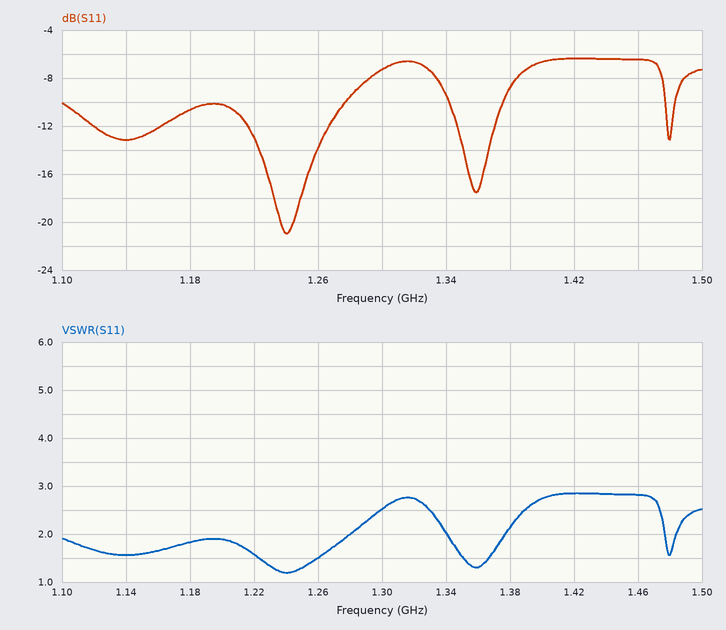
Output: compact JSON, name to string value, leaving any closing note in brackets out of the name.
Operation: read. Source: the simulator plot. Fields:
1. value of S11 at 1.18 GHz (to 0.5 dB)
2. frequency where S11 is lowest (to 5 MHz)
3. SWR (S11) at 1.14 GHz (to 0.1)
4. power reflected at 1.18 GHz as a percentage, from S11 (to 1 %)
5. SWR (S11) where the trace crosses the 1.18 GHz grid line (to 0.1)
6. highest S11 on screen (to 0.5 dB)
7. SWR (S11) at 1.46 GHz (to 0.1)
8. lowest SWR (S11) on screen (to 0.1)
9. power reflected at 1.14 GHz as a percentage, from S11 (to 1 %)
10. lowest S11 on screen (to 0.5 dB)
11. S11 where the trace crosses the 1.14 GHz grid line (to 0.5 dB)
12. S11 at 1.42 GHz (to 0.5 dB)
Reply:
{"value of S11 at 1.18 GHz": "-10.5 dB", "frequency where S11 is lowest": "1.240 GHz", "SWR (S11) at 1.14 GHz": "1.6", "power reflected at 1.18 GHz as a percentage, from S11": "9 %", "SWR (S11) where the trace crosses the 1.18 GHz grid line": "1.8", "highest S11 on screen": "-6.5 dB", "SWR (S11) at 1.46 GHz": "2.8", "lowest SWR (S11) on screen": "1.2", "power reflected at 1.14 GHz as a percentage, from S11": "5 %", "lowest S11 on screen": "-21.0 dB", "S11 where the trace crosses the 1.14 GHz grid line": "-13.0 dB", "S11 at 1.42 GHz": "-6.5 dB"}
